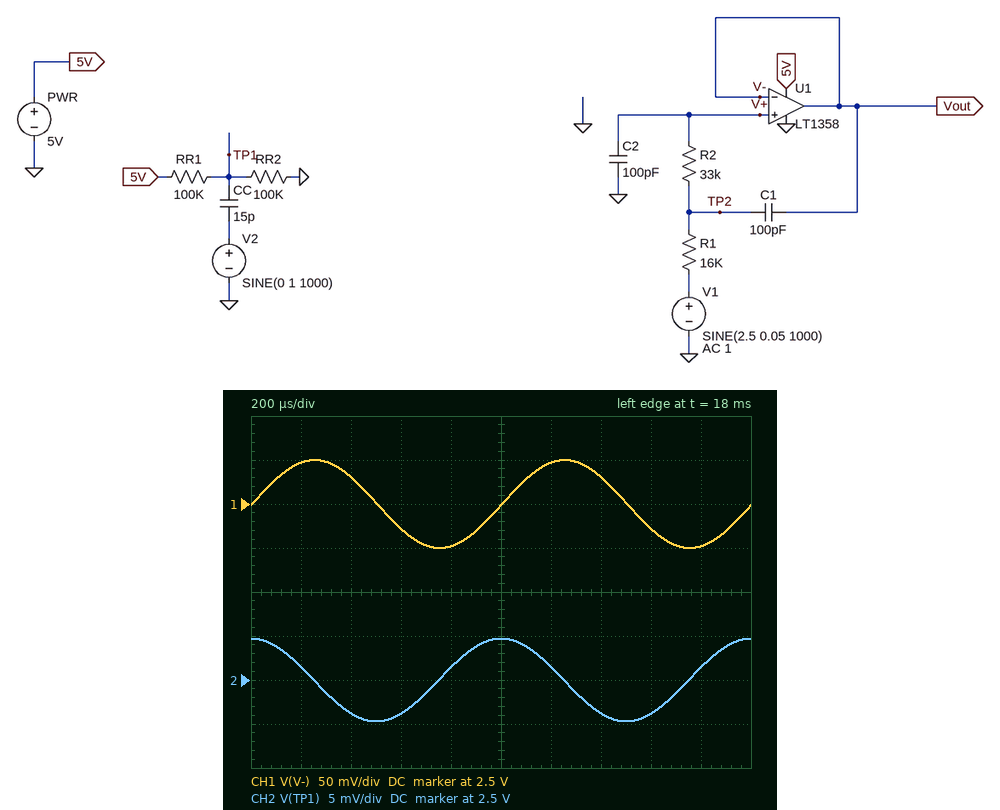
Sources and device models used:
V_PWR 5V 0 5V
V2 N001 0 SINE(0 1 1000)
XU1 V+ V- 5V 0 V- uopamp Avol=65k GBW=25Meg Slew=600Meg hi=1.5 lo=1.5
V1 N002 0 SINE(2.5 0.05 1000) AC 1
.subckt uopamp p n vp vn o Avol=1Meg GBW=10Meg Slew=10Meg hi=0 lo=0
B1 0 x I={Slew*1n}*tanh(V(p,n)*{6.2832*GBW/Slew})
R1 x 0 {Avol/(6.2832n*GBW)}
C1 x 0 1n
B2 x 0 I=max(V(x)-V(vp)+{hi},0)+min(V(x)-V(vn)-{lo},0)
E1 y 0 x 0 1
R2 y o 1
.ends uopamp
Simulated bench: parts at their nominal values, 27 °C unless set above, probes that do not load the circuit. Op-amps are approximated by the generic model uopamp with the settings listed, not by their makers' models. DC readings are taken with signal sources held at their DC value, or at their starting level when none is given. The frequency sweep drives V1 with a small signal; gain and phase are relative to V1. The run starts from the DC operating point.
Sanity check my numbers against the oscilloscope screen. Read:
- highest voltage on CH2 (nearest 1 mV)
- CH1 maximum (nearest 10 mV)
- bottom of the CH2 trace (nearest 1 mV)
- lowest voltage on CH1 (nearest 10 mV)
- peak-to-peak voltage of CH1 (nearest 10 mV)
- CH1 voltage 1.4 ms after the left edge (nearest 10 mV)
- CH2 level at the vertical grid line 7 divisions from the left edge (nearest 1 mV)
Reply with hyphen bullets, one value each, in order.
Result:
- 2.505 V
- 2.55 V
- 2.495 V
- 2.45 V
- 100 mV
- 2.53 V
- 2.496 V
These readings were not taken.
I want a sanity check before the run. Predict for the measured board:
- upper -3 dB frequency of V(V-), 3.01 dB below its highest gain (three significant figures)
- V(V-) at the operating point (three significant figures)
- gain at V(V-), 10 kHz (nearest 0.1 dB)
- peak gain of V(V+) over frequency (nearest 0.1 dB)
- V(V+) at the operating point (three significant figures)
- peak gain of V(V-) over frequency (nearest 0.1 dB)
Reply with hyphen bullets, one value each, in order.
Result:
- 40.7 kHz
- 2.50 V
- -0.2 dB
- 0 dB
- 2.50 V
- 0 dB
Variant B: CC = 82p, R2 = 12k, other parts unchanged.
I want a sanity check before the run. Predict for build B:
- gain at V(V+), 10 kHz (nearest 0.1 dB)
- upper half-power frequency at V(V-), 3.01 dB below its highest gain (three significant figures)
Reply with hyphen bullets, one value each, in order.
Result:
- -0.1 dB
- 72.9 kHz
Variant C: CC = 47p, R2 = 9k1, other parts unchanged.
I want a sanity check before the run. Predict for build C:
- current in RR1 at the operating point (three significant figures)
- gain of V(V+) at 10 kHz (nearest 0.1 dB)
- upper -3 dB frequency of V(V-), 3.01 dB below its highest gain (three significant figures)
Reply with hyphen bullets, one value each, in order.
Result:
- 25.0 µA
- -0.1 dB
- 80.4 kHz
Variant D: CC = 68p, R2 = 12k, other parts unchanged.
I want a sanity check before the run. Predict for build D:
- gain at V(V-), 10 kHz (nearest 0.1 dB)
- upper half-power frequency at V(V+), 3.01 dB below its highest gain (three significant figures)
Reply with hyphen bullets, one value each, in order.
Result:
- -0.1 dB
- 72.9 kHz
